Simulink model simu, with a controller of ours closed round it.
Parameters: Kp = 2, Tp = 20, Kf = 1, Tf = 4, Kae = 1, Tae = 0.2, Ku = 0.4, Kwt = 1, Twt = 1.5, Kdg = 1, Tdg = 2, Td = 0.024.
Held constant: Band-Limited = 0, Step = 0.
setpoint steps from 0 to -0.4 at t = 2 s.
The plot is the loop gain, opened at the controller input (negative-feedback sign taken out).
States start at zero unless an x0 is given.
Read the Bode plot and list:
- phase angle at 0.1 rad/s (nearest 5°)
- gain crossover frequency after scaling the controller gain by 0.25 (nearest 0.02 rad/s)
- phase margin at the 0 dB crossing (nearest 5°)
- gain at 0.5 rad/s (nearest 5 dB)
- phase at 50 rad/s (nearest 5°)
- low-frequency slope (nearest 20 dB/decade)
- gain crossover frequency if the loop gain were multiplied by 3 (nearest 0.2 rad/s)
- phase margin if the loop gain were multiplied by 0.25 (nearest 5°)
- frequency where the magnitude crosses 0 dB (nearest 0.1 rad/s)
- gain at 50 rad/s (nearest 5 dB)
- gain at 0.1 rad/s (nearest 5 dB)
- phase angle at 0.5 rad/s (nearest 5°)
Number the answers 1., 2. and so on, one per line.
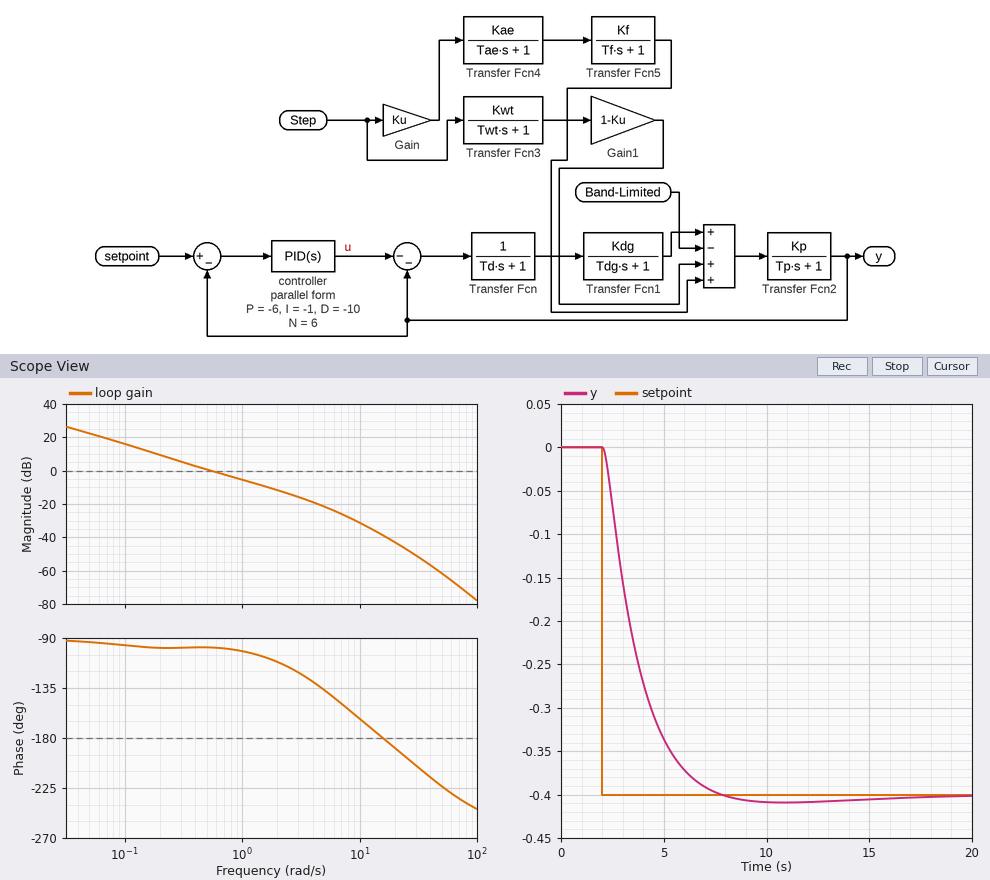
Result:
1. -95°
2. 0.16 rad/s
3. 80°
4. 0 dB
5. -225°
6. -20 dB/decade
7. 1.6 rad/s
8. 80°
9. 0.5 rad/s
10. -60 dB
11. 15 dB
12. -100°
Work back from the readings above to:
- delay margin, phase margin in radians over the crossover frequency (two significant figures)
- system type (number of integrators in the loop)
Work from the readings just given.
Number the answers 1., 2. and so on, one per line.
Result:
1. 2.8 s
2. 1
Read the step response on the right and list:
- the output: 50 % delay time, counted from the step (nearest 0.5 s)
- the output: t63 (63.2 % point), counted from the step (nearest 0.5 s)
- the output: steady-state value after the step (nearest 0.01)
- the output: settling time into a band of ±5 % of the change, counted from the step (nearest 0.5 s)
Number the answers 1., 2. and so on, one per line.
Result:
1. 1.5 s
2. 2.0 s
3. -0.40
4. 4.5 s
